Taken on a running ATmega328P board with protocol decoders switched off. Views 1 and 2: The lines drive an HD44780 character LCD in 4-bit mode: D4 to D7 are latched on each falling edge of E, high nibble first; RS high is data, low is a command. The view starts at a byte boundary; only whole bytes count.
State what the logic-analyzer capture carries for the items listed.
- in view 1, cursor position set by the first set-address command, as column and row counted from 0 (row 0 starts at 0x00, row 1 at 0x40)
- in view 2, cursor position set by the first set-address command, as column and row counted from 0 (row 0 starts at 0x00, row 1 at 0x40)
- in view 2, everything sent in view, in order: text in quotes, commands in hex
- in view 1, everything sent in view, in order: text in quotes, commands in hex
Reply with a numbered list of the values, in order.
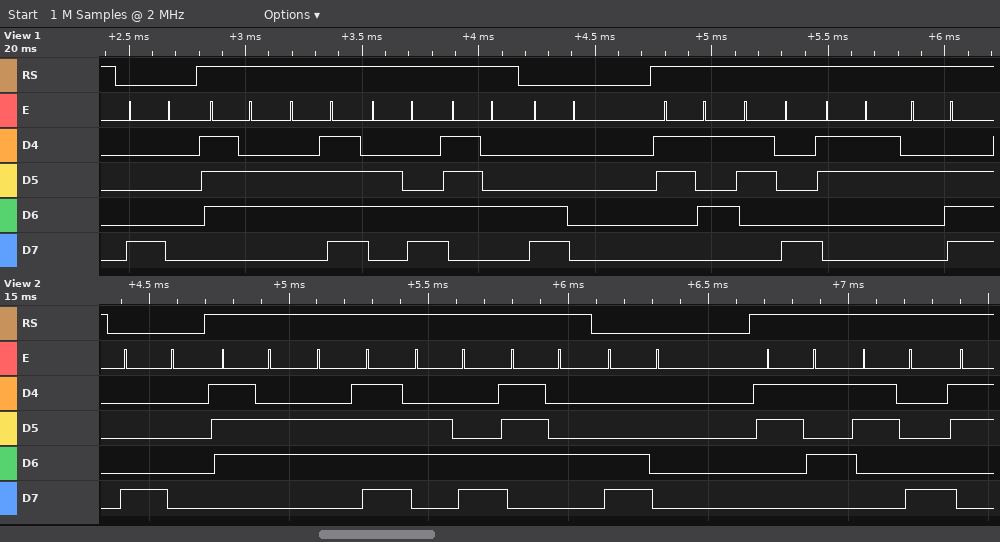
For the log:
1. column 0, row 0
2. column 0, row 0
3. 0x80 "volt" 0xC0 "58"
4. 0x80 "volt" 0xC0 "583."
